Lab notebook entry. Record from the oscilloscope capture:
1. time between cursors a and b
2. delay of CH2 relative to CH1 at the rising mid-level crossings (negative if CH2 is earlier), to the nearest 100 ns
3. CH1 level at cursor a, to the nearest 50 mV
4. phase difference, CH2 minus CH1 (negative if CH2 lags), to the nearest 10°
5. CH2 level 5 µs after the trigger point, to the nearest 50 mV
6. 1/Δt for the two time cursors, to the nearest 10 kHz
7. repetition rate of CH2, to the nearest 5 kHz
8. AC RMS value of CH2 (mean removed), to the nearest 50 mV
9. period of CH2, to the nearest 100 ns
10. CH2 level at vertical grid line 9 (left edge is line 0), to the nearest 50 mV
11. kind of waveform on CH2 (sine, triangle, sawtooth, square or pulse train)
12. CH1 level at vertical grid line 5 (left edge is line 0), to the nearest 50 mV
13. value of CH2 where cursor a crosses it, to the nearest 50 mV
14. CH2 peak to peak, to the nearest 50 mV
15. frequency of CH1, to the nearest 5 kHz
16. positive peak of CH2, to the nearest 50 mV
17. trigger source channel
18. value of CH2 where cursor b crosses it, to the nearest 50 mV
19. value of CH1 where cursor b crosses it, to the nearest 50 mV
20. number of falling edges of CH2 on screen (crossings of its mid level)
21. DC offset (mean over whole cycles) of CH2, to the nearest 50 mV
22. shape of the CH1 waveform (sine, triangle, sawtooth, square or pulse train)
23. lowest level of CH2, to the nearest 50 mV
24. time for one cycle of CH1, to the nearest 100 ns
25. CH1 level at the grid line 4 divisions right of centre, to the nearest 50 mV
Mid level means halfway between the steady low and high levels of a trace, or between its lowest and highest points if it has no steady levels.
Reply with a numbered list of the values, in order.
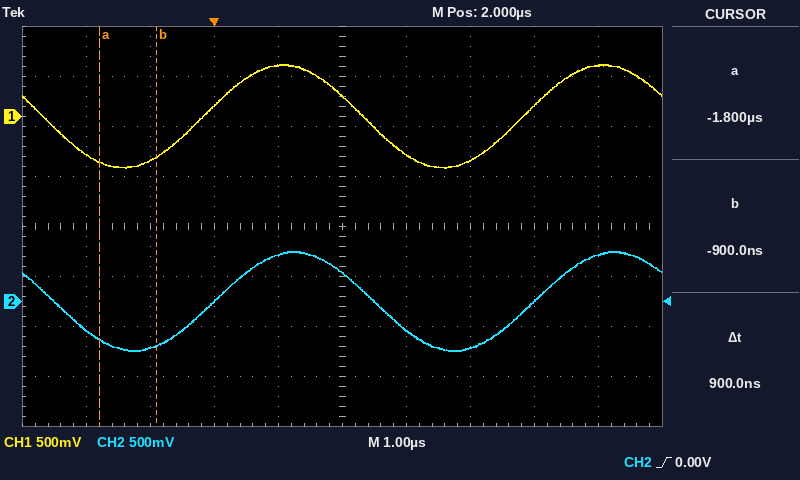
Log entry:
1. 900 ns
2. +200 ns
3. -450 mV
4. -10°
5. 0 mV
6. 1.11 MHz
7. 200 kHz
8. 350 mV
9. 5.0 µs
10. 450 mV
11. sine
12. 200 mV
13. -400 mV
14. 1.00 V
15. 200 kHz
16. 500 mV
17. CH2
18. -450 mV
19. -400 mV
20. 2
21. 0 mV
22. sine
23. -500 mV
24. 5.0 µs
25. 500 mV
